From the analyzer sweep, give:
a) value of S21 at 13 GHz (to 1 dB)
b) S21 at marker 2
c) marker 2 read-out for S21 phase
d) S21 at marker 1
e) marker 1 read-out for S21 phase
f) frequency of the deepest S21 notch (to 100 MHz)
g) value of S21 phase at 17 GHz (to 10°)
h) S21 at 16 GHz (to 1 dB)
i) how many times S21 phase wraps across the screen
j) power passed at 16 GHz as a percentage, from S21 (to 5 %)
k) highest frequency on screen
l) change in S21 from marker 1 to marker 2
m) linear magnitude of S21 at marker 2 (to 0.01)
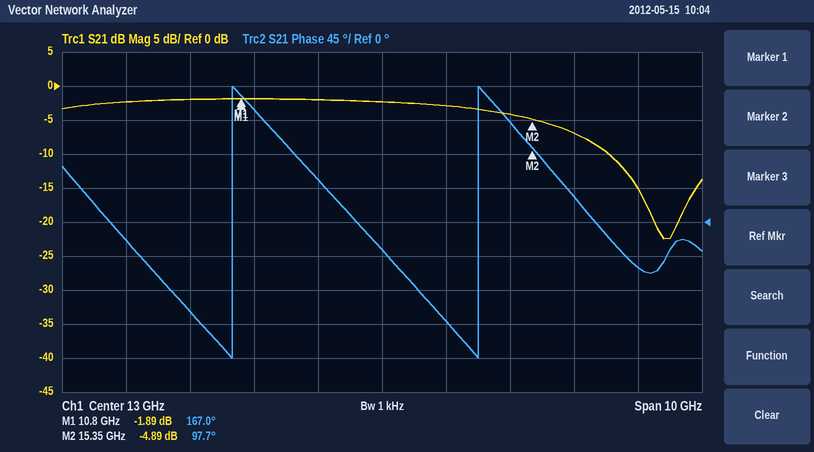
-2 dB
-4.89 dB
97.7°
-1.89 dB
167.0°
17.4 GHz
-60°
-7 dB
2
20 %
18 GHz
-3.00 dB
0.57
